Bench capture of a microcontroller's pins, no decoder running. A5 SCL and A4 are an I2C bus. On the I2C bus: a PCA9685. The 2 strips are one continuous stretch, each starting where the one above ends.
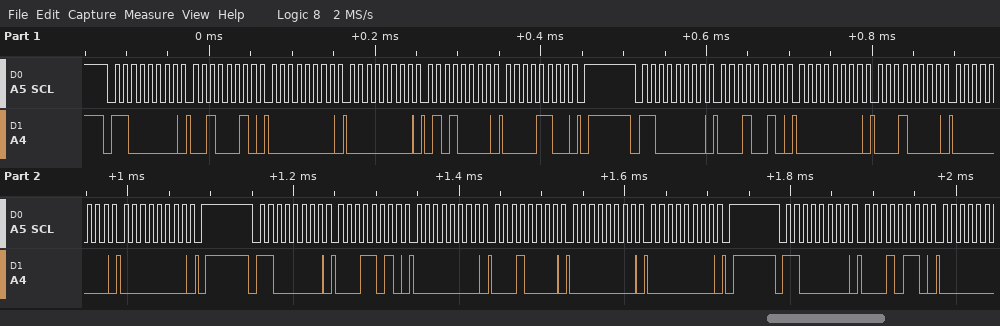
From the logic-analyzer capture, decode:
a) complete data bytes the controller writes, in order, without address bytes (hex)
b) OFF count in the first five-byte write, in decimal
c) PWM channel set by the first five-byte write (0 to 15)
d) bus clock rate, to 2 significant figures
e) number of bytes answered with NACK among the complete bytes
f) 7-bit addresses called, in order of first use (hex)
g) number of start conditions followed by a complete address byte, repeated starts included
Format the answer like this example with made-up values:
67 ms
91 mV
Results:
22 00 00 50 0C 12 00 10 00 00 1A 00 10 00 00 16
3152
7
100 kHz
0
0x60
4
